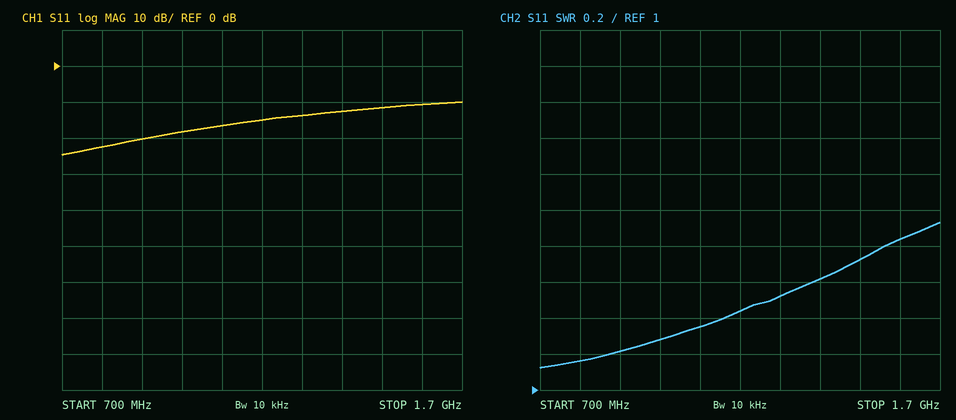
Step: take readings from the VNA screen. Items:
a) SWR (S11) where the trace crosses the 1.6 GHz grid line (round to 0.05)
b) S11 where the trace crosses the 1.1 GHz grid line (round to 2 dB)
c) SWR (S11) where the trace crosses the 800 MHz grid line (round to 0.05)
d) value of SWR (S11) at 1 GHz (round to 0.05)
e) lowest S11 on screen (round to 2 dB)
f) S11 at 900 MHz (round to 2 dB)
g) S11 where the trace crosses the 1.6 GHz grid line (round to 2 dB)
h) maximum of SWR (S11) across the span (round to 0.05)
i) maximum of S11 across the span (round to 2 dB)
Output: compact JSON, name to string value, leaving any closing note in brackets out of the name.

{"SWR (S11) where the trace crosses the 1.6 GHz grid line": "1.85", "S11 where the trace crosses the 1.1 GHz grid line": "-16 dB", "SWR (S11) where the trace crosses the 800 MHz grid line": "1.15", "value of SWR (S11) at 1 GHz": "1.30", "lowest S11 on screen": "-24 dB", "S11 at 900 MHz": "-20 dB", "S11 where the trace crosses the 1.6 GHz grid line": "-10 dB", "maximum of SWR (S11) across the span": "1.95", "maximum of S11 across the span": "-10 dB"}
